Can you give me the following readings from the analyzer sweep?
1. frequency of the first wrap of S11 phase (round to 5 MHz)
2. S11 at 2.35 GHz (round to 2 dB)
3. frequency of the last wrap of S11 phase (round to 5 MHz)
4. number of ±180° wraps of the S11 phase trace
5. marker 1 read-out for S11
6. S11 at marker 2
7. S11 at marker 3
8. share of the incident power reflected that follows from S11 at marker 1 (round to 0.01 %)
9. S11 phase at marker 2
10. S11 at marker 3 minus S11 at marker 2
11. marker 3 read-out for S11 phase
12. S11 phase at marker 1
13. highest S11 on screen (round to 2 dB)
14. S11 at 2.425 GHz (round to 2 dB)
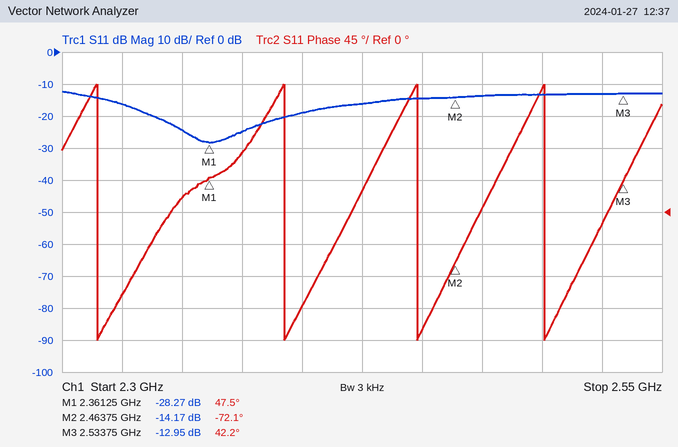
2.315 GHz
-24 dB
2.500 GHz
4
-28.27 dB
-14.17 dB
-12.95 dB
0.15 %
-72.1°
1.22 dB
42.2°
47.5°
-12 dB
-16 dB
